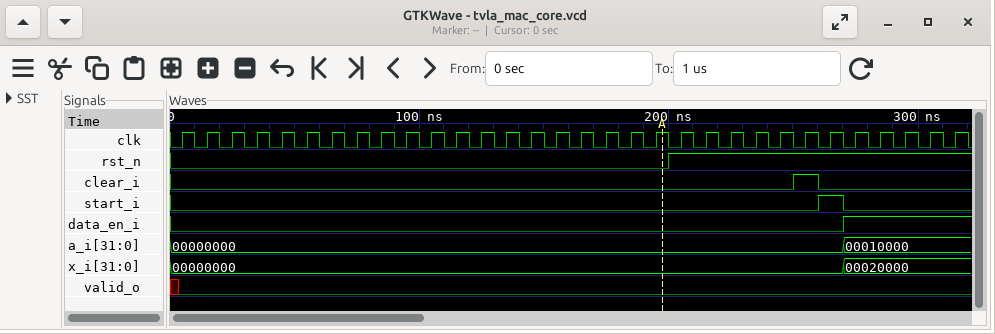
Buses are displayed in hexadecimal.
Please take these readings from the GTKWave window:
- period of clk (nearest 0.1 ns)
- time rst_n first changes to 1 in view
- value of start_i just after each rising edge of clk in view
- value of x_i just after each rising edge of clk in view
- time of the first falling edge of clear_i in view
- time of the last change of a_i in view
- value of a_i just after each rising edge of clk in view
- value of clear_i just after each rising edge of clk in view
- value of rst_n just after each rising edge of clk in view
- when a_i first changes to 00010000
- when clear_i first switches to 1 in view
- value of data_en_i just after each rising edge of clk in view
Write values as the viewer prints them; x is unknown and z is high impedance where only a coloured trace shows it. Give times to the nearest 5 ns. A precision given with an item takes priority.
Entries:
10 ns
200 ns
0 0 0 0 0 0 0 0 0 0 0 0 0 0 0 0 0 0 0 0 0 0 0 0 0 0 1 0 0 0 0 0
00000000, 00000000, 00000000, 00000000, 00000000, 00000000, 00000000, 00000000, 00000000, 00000000, 00000000, 00000000, 00000000, 00000000, 00000000, 00000000, 00000000, 00000000, 00000000, 00000000, 00000000, 00000000, 00000000, 00000000, 00000000, 00000000, 00000000, 00020000, 00020000, 00020000, 00020000, 00020000
260 ns
270 ns
00000000, 00000000, 00000000, 00000000, 00000000, 00000000, 00000000, 00000000, 00000000, 00000000, 00000000, 00000000, 00000000, 00000000, 00000000, 00000000, 00000000, 00000000, 00000000, 00000000, 00000000, 00000000, 00000000, 00000000, 00000000, 00000000, 00000000, 00010000, 00010000, 00010000, 00010000, 00010000
0 0 0 0 0 0 0 0 0 0 0 0 0 0 0 0 0 0 0 0 0 0 0 0 0 1 0 0 0 0 0 0
0 0 0 0 0 0 0 0 0 0 0 0 0 0 0 0 0 0 0 0 1 1 1 1 1 1 1 1 1 1 1 1
270 ns
250 ns
0 0 0 0 0 0 0 0 0 0 0 0 0 0 0 0 0 0 0 0 0 0 0 0 0 0 0 1 1 1 1 1
